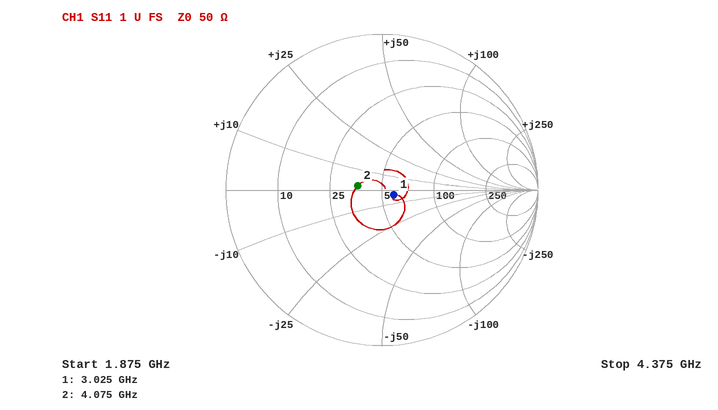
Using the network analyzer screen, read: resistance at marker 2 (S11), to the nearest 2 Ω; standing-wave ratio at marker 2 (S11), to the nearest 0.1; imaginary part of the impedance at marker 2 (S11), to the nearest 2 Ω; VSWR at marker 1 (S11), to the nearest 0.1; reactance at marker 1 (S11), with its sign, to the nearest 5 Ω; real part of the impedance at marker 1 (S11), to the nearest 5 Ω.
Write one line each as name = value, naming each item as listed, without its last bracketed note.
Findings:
resistance at marker 2 (S11), to the nearest 2 Ω = 36 Ω
standing-wave ratio at marker 2 (S11), to the nearest 0.1 = 1.4
imaginary part of the impedance at marker 2 (S11), to the nearest 2 Ω = +2 Ω
VSWR at marker 1 (S11), to the nearest 0.1 = 1.2
reactance at marker 1 (S11), with its sign, to the nearest 5 Ω = -5 Ω
real part of the impedance at marker 1 (S11), to the nearest 5 Ω = 60 Ω
